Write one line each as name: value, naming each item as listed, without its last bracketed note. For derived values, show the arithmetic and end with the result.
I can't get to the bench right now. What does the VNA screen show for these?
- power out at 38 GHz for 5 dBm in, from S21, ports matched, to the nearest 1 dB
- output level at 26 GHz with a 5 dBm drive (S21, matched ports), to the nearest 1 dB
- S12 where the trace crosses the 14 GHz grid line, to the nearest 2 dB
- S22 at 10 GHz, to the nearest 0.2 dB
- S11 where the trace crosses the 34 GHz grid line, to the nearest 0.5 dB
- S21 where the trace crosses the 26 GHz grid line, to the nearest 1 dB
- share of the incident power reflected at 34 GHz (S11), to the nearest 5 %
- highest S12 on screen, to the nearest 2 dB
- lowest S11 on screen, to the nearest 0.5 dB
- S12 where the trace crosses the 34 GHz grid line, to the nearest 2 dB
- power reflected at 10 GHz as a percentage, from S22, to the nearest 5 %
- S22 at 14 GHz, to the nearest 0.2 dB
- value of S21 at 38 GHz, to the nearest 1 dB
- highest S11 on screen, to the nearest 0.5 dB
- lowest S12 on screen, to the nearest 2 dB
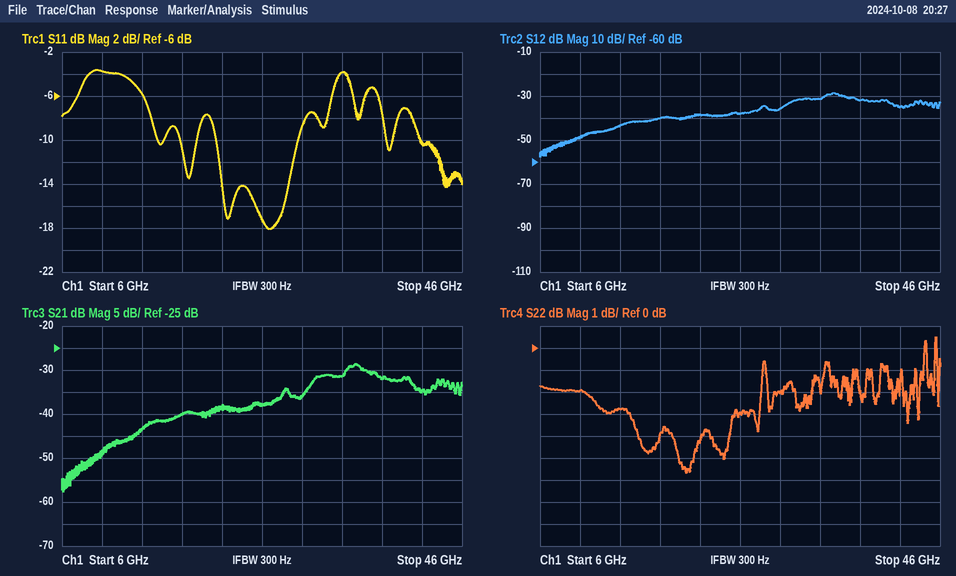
power out at 38 GHz for 5 dBm in, from S21, ports matched, to the nearest 1 dB: 5 dBm + (-32 dB) = -27 dBm
output level at 26 GHz with a 5 dBm drive (S21, matched ports), to the nearest 1 dB: 5 dBm + (-38 dB) = -33 dBm
S12 where the trace crosses the 14 GHz grid line, to the nearest 2 dB: -44 dB
S22 at 10 GHz, to the nearest 0.2 dB: -2.0 dB
S11 where the trace crosses the 34 GHz grid line, to the nearest 0.5 dB: -4.0 dB
S21 where the trace crosses the 26 GHz grid line, to the nearest 1 dB: -38 dB
share of the incident power reflected at 34 GHz (S11), to the nearest 5 %: 10^(-4/10) ≈ 40 %
highest S12 on screen, to the nearest 2 dB: -28 dB
lowest S11 on screen, to the nearest 0.5 dB: -18.0 dB
S12 where the trace crosses the 34 GHz grid line, to the nearest 2 dB: -32 dB
power reflected at 10 GHz as a percentage, from S22, to the nearest 5 %: 10^(-2/10) ≈ 63.1 %, so 65 % to the nearest 5 %
S22 at 14 GHz, to the nearest 0.2 dB: -2.8 dB
value of S21 at 38 GHz, to the nearest 1 dB: -32 dB
highest S11 on screen, to the nearest 0.5 dB: -3.5 dB
lowest S12 on screen, to the nearest 2 dB: -58 dB
